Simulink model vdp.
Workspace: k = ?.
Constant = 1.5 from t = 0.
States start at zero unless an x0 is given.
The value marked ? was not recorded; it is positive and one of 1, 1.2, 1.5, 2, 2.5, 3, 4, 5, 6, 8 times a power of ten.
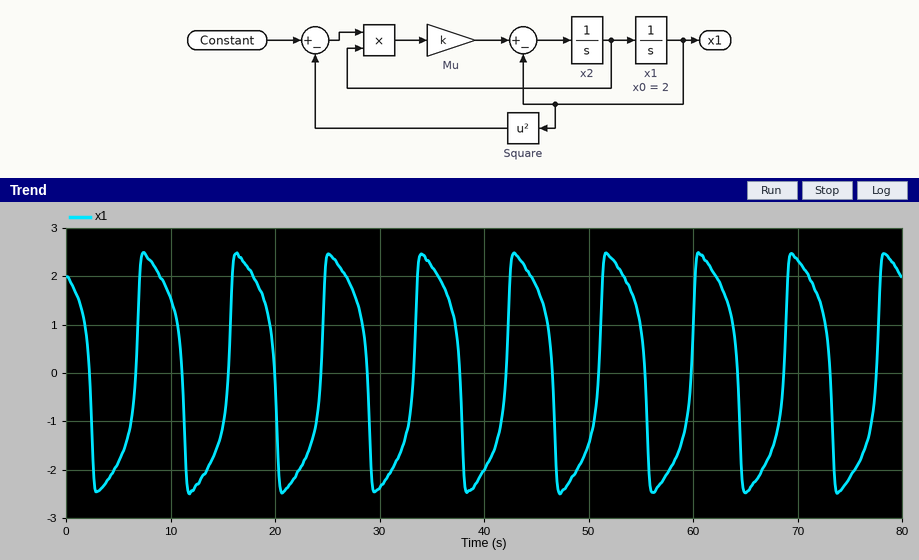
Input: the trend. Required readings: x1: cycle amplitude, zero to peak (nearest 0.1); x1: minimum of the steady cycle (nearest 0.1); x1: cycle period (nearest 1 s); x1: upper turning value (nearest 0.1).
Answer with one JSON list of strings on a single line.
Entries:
["2.5", "-2.5", "9 s", "2.5"]
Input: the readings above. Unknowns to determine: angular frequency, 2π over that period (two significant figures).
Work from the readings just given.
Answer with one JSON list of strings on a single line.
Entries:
["0.70 rad/s"]
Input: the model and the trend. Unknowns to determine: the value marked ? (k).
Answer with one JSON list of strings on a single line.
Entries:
["2"]
